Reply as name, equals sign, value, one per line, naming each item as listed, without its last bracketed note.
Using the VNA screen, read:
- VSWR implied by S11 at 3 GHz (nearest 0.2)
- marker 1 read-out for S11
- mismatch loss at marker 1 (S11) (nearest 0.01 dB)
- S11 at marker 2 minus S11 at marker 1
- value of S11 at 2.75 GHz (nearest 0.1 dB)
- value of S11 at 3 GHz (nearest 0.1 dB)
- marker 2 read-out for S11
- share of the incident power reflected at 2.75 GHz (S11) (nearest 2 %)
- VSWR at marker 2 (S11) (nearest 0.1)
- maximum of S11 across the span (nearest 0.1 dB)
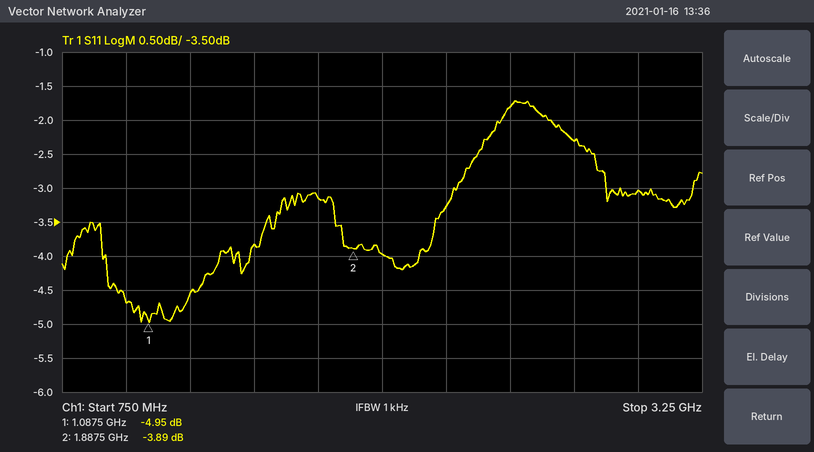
VSWR implied by S11 at 3 GHz = 5.8
marker 1 read-out for S11 = -4.95 dB
mismatch loss at marker 1 (S11) = 1.67 dB
S11 at marker 2 minus S11 at marker 1 = 1.06 dB
value of S11 at 2.75 GHz = -2.3 dB
value of S11 at 3 GHz = -3.0 dB
marker 2 read-out for S11 = -3.89 dB
share of the incident power reflected at 2.75 GHz (S11) = 58 %
VSWR at marker 2 (S11) = 4.5
maximum of S11 across the span = -1.7 dB
